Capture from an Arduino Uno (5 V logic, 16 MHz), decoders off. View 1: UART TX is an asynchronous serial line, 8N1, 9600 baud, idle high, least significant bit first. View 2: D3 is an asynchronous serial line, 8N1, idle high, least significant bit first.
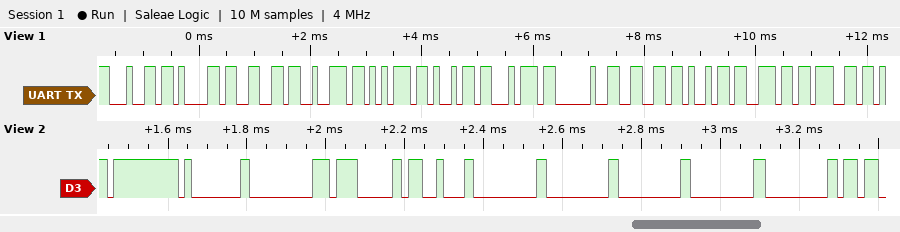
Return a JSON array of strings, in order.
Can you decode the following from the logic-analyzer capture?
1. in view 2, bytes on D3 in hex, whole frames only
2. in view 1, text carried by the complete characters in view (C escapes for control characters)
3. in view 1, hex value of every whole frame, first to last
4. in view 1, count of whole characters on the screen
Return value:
["FF 01 00 07 13 00 00 00 00 00", "\"dafruit fing\"", "0x64 0x61 0x66 0x72 0x75 0x69 0x74 0x20 0x66 0x69 0x6E 0x67", "12"]
